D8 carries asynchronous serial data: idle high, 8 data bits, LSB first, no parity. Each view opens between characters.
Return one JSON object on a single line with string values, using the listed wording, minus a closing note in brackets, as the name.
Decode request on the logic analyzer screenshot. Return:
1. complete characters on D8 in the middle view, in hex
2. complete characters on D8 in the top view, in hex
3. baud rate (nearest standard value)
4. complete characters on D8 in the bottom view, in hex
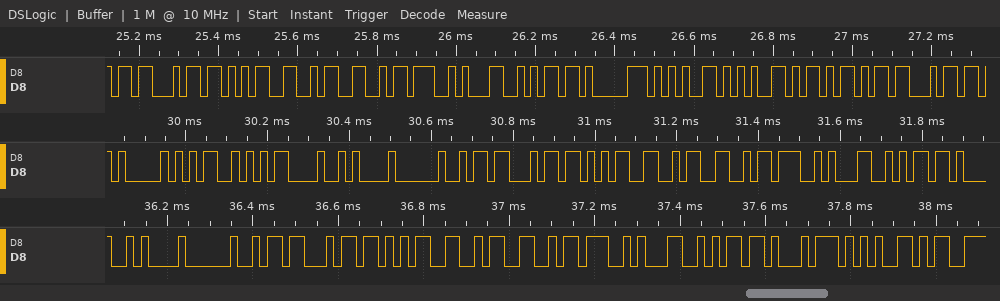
{"complete characters on D8 in the middle view, in hex": "41, 4D, 0D, 0A, 20, 1B, 5B, 33, 33, 3B, 31, 6D", "complete characters on D8 in the top view, in hex": "1B, 5B, 33, 33, 3B, 31, 6D, 70, 65, 65, 6B, 1B", "baud rate": "57600 baud", "complete characters on D8 in the bottom view, in hex": "0A, 20, 1B, 5B, 33, 33, 3B, 31, 6D, 74, 65"}
